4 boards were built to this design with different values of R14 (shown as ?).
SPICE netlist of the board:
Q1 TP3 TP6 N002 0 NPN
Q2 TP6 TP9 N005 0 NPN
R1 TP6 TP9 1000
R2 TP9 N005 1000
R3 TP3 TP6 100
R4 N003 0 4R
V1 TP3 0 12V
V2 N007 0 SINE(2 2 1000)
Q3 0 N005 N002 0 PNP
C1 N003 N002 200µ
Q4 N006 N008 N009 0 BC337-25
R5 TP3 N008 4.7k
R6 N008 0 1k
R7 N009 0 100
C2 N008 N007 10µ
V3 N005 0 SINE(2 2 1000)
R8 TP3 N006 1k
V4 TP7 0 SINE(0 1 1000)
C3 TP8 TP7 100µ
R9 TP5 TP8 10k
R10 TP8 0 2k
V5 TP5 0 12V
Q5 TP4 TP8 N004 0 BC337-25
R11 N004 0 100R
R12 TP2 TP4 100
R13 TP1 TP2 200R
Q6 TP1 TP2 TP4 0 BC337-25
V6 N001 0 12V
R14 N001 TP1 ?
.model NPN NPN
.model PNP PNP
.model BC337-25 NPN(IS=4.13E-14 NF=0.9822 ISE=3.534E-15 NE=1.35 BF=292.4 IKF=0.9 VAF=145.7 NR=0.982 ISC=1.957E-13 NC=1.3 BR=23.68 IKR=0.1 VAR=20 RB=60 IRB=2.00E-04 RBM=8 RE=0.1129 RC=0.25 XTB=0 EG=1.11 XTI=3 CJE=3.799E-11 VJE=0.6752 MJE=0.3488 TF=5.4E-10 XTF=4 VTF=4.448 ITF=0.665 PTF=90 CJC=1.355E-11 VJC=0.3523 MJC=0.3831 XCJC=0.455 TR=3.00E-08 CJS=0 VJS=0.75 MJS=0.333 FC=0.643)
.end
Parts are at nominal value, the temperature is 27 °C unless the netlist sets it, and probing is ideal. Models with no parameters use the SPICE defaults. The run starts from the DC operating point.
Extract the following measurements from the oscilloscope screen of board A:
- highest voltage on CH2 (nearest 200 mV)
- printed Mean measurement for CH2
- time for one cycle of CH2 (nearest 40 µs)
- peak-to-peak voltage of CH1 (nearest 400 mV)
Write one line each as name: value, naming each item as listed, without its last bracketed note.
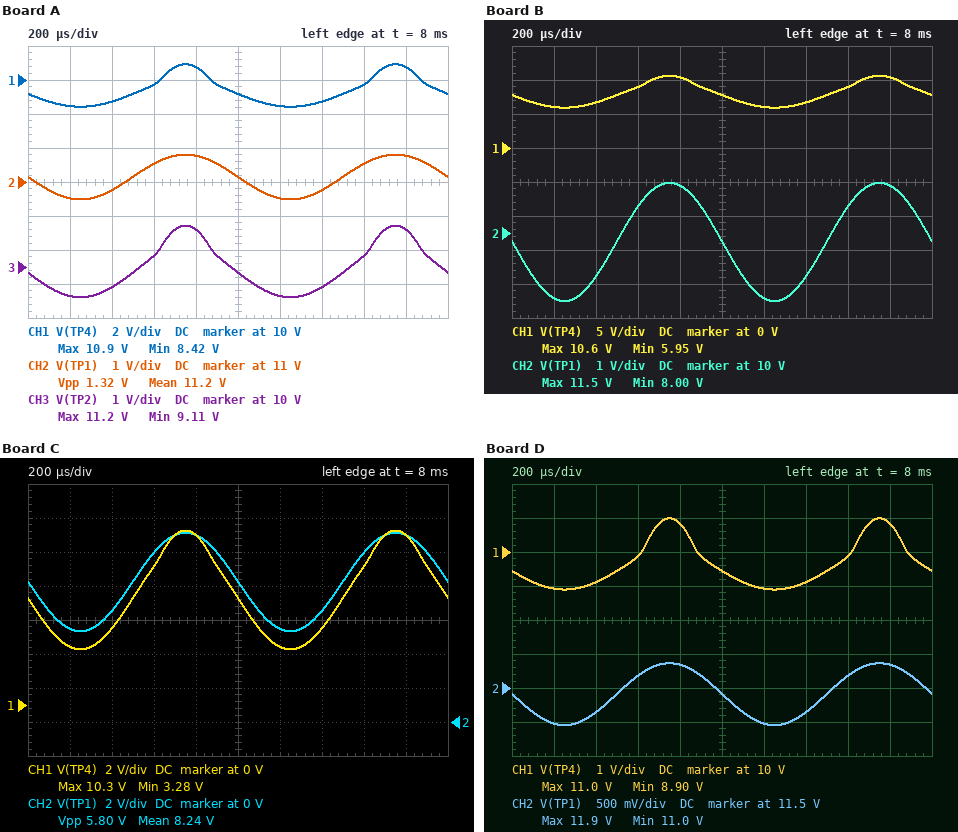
highest voltage on CH2: 11.8 V
printed Mean measurement for CH2: 11.2 V
time for one cycle of CH2: 1.00 ms
peak-to-peak voltage of CH1: 2.4 V
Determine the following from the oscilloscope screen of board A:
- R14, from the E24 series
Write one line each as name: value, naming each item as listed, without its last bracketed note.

R14, from the E24 series: 68 Ω
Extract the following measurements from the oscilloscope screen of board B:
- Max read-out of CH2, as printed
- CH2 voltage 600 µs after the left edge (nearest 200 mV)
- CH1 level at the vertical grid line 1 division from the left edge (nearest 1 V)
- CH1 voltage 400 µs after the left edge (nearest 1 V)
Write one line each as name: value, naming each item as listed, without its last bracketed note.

Max read-out of CH2, as printed: 11.5 V
CH2 voltage 600 µs after the left edge: 10.8 V
CH1 level at the vertical grid line 1 division from the left edge: 6 V
CH1 voltage 400 µs after the left edge: 7 V
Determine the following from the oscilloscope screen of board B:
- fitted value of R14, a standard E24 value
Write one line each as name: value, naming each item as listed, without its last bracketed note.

fitted value of R14, a standard E24 value: 180 Ω
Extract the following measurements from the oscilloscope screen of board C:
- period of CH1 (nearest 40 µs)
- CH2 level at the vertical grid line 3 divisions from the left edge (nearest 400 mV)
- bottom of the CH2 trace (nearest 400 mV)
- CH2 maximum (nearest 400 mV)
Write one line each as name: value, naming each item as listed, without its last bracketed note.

period of CH1: 1.00 ms
CH2 level at the vertical grid line 3 divisions from the left edge: 10.0 V
bottom of the CH2 trace: 5.2 V
CH2 maximum: 11.2 V
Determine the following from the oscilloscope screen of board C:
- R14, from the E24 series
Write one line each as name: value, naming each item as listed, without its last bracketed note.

R14, from the E24 series: 300 Ω
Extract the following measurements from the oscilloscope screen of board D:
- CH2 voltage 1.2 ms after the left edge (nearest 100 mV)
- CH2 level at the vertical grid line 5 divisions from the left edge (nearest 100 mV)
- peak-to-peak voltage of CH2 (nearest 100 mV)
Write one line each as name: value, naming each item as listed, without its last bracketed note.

CH2 voltage 1.2 ms after the left edge: 11.0 V
CH2 level at the vertical grid line 5 divisions from the left edge: 11.4 V
peak-to-peak voltage of CH2: 900 mV
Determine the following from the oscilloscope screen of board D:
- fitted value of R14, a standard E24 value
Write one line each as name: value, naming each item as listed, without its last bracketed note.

fitted value of R14, a standard E24 value: 47 Ω
